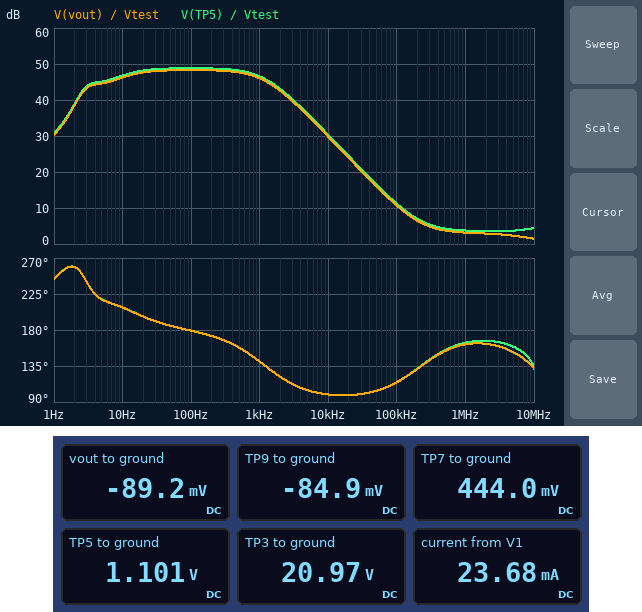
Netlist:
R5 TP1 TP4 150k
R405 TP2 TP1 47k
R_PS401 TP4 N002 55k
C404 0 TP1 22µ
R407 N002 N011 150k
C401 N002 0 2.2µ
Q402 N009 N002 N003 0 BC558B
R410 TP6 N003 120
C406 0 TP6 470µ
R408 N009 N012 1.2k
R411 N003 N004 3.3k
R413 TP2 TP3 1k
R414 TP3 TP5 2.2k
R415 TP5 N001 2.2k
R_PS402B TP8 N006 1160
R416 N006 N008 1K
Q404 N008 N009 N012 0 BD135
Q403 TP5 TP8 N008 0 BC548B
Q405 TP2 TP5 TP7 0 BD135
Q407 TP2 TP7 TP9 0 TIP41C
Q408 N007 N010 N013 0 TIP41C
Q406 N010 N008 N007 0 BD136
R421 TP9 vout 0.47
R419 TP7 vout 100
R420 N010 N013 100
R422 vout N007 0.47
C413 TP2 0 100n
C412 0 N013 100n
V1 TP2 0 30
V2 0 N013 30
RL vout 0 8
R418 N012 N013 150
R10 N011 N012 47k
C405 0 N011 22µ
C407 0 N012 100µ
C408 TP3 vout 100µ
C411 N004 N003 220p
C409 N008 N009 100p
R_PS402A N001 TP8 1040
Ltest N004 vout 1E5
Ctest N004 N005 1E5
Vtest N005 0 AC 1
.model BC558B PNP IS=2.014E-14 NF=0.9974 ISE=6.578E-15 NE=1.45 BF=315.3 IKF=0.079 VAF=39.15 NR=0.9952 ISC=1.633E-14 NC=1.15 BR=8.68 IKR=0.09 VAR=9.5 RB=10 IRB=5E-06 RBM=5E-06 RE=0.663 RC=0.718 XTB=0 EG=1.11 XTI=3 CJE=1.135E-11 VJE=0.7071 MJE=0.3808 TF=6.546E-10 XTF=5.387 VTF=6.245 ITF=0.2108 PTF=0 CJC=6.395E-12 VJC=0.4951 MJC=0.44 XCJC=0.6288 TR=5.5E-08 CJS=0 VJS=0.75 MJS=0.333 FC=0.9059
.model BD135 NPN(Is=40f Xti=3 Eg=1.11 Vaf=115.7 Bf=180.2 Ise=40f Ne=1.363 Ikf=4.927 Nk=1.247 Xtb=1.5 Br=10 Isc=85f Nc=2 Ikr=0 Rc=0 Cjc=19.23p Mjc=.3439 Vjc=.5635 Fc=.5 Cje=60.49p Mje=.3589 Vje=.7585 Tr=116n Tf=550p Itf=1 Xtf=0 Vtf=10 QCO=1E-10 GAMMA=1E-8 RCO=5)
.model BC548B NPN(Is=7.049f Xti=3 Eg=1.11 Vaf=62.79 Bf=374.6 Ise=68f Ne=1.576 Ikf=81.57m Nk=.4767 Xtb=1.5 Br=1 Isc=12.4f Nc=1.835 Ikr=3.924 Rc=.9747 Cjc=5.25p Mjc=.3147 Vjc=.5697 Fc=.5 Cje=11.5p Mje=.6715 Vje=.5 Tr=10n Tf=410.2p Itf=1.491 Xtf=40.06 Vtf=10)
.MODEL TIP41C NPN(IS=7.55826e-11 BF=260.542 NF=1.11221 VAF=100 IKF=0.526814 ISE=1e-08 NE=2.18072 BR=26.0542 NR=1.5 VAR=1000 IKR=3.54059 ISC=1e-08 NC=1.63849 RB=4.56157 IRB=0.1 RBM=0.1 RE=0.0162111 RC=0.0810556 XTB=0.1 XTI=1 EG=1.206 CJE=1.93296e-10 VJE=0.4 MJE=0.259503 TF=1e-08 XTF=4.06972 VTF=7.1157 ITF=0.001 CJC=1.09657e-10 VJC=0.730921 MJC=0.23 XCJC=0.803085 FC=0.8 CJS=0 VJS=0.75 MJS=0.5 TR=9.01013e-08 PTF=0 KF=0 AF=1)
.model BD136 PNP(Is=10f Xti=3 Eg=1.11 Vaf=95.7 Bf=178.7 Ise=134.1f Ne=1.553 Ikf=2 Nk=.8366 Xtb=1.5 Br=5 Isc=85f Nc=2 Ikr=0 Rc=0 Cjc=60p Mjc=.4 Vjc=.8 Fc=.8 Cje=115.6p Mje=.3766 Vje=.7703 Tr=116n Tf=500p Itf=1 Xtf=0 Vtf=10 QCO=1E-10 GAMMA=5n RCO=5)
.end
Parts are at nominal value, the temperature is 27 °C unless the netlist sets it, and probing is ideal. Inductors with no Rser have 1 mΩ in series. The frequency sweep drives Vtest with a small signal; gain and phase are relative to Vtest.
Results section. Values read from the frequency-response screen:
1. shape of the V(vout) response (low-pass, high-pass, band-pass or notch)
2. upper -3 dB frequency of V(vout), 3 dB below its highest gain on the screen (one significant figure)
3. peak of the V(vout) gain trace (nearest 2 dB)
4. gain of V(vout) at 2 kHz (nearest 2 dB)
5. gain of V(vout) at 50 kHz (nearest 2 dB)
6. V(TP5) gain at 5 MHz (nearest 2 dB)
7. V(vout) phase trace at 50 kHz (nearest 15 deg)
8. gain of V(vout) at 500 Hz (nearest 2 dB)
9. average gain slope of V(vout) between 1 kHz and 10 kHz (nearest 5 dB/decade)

band-pass
1 kHz
48 dB
42 dB
16 dB
4 dB
105 deg
48 dB
-15 dB/decade
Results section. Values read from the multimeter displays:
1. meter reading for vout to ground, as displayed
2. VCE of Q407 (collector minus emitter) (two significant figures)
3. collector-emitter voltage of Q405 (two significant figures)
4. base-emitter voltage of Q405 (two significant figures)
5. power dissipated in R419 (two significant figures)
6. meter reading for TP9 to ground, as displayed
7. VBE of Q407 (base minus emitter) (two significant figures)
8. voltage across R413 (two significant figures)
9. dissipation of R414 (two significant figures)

-89.2 mV
30 V
30 V
660 mV
2.8 mW
-84.9 mV
530 mV
9.0 V
180 mW
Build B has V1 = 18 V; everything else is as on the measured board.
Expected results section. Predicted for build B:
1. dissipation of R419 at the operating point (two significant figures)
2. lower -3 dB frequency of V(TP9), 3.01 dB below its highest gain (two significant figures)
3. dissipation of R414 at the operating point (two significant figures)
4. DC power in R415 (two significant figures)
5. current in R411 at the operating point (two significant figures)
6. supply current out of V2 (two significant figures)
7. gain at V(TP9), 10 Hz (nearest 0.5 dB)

340 µW
8.7 Hz
110 mW
270 µW
600 µA
700 mA
46.0 dB
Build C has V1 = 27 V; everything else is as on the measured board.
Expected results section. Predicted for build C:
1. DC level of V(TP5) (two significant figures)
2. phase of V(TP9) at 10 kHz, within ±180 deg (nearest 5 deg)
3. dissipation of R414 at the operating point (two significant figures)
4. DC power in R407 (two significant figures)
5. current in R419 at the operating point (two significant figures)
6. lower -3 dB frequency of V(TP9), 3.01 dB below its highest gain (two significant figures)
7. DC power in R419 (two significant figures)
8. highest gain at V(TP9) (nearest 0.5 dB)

-350 mV
100 deg
160 mW
2.3 mW
4.5 mA
8.0 Hz
2.0 mW
49.0 dB
